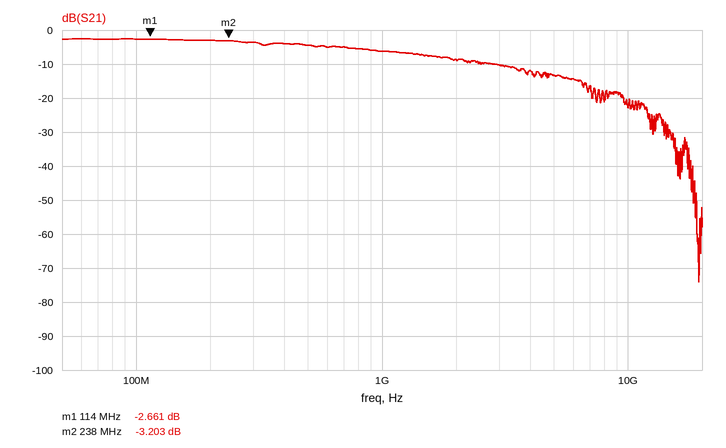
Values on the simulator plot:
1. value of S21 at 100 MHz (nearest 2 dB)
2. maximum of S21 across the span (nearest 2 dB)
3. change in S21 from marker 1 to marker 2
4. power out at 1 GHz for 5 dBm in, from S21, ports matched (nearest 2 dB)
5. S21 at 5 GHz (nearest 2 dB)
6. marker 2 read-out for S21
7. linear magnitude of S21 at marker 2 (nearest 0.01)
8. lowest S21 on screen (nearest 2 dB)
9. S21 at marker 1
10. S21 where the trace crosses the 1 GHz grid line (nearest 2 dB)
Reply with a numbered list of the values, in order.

1. -2 dB
2. -2 dB
3. -0.542 dB
4. -2 dBm
5. -14 dB
6. -3.203 dB
7. 0.69
8. -74 dB
9. -2.661 dB
10. -6 dB
